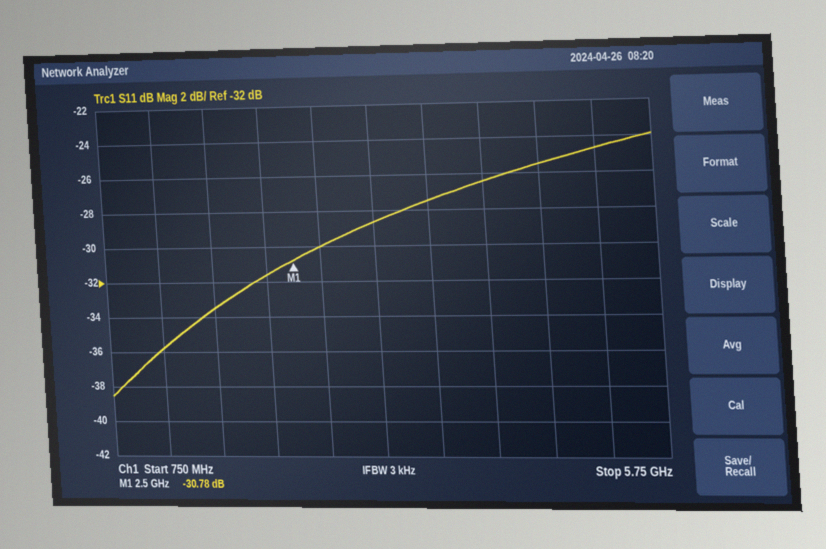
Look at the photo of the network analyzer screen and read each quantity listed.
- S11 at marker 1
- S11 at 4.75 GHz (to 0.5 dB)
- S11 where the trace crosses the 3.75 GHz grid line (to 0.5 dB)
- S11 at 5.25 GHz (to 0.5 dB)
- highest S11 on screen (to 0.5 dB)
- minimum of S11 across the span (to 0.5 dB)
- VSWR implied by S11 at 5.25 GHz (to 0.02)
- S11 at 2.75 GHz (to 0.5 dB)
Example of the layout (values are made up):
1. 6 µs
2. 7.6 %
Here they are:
1. -30.78 dB
2. -25.5 dB
3. -27.5 dB
4. -24.5 dB
5. -24.0 dB
6. -38.5 dB
7. 1.12
8. -30.0 dB
